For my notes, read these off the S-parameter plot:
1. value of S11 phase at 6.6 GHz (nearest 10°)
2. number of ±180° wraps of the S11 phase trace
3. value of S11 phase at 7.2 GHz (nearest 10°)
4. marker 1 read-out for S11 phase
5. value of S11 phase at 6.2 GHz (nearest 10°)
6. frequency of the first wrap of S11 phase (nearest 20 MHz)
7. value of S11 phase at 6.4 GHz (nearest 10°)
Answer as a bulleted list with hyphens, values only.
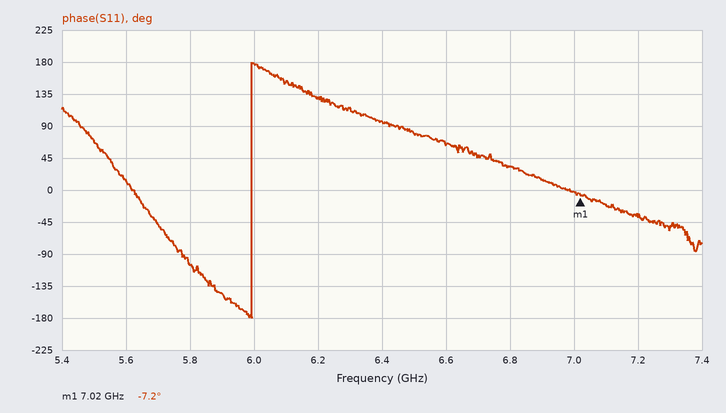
- 60°
- 1
- -40°
- -7.2°
- 130°
- 6.00 GHz
- 100°
